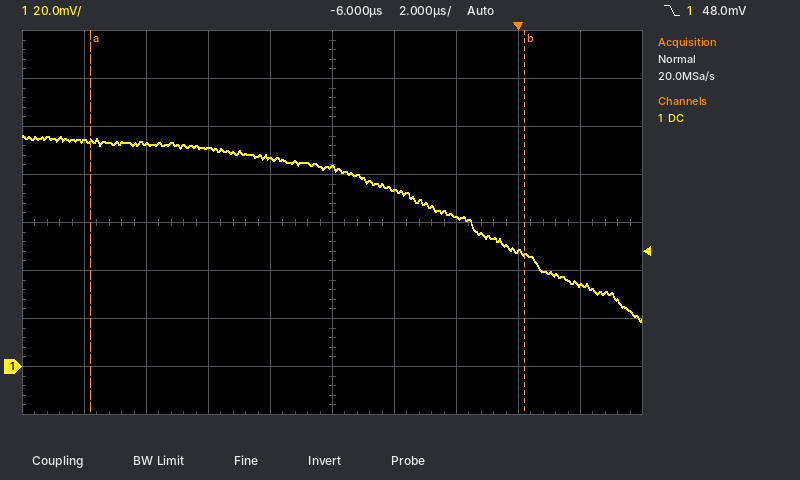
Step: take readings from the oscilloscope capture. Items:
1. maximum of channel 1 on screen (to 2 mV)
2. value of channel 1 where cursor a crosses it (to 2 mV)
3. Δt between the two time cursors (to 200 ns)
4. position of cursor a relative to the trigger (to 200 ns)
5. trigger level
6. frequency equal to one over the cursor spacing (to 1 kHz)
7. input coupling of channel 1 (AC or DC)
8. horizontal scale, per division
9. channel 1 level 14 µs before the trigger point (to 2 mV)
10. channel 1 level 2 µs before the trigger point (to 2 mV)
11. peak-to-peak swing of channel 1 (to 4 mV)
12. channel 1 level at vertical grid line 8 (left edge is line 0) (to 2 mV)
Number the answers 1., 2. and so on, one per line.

1. 96 mV
2. 94 mV
3. 14.0 µs
4. -13.8 µs
5. 48.0 mV
6. 71 kHz
7. DC
8. 2 µs
9. 94 mV
10. 62 mV
11. 76 mV
12. 48 mV
